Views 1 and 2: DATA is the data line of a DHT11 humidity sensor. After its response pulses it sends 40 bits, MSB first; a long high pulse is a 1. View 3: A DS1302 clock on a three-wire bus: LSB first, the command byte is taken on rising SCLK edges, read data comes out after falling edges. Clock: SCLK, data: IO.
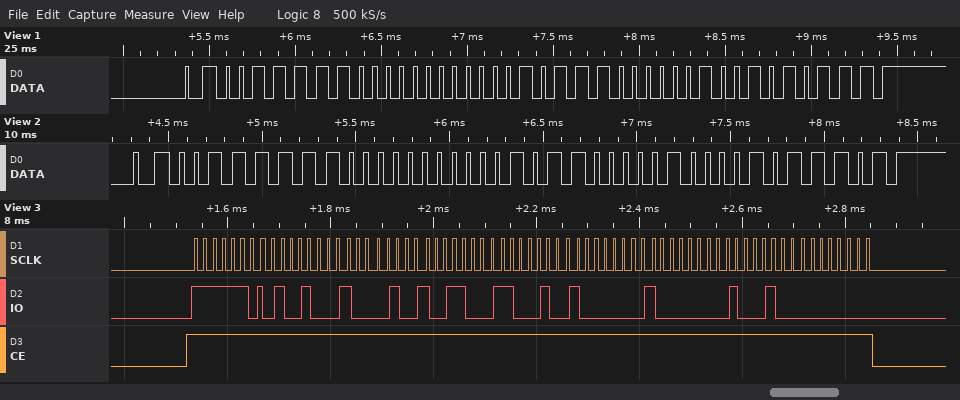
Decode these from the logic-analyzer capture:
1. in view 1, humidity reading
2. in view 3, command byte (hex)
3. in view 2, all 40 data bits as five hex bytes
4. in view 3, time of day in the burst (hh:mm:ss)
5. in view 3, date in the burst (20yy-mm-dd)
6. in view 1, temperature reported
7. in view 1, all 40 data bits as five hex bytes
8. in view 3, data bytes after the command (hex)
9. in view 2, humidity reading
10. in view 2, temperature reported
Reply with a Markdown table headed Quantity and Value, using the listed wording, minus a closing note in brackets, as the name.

| Quantity | Value |
|---|---|
| in view 1, humidity reading | 62 % |
| in view 3, command byte | 0xBF |
| in view 2, all 40 data bits as five hex bytes | 3F 00 16 08 5D |
| in view 3, time of day in the burst | 19:21:12 |
| in view 3, date in the burst | 2022-01-23 |
| in view 1, temperature reported | 23.2 °C |
| in view 1, all 40 data bits as five hex bytes | 3E 00 17 02 57 |
| in view 3, data bytes after the command | 12 21 19 23 01 01 22 00 |
| in view 2, humidity reading | 63 % |
| in view 2, temperature reported | 22.8 °C |
